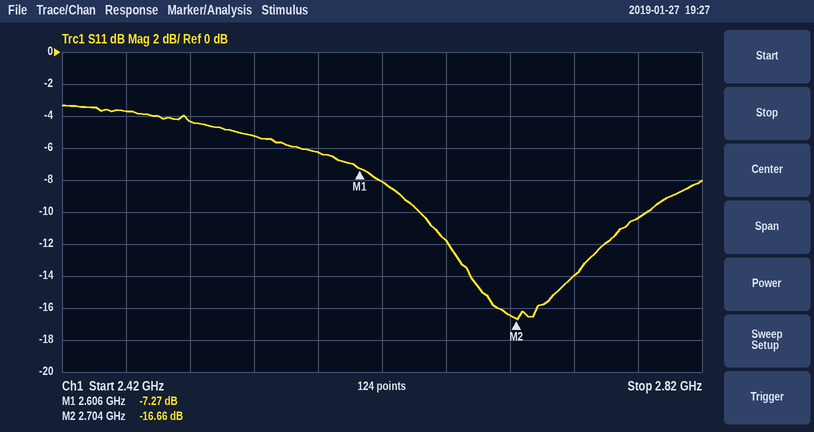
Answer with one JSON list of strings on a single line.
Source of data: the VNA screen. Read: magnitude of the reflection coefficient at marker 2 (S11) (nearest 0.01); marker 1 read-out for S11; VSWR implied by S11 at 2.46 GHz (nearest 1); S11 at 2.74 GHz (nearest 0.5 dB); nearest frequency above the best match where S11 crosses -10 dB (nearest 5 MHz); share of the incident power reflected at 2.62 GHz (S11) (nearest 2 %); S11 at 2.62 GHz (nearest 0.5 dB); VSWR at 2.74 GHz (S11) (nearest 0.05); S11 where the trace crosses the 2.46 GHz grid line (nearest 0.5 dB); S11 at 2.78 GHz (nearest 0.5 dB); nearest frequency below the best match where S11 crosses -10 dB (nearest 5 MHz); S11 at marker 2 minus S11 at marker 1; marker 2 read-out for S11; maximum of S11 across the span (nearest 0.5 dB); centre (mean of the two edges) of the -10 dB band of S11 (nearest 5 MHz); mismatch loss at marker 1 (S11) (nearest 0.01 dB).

["0.15", "-7.27 dB", "5", "-14.0 dB", "2.785 GHz", "16 %", "-8.0 dB", "1.50", "-3.5 dB", "-10.5 dB", "2.645 GHz", "-9.39 dB", "-16.66 dB", "-3.5 dB", "2.715 GHz", "0.90 dB"]
